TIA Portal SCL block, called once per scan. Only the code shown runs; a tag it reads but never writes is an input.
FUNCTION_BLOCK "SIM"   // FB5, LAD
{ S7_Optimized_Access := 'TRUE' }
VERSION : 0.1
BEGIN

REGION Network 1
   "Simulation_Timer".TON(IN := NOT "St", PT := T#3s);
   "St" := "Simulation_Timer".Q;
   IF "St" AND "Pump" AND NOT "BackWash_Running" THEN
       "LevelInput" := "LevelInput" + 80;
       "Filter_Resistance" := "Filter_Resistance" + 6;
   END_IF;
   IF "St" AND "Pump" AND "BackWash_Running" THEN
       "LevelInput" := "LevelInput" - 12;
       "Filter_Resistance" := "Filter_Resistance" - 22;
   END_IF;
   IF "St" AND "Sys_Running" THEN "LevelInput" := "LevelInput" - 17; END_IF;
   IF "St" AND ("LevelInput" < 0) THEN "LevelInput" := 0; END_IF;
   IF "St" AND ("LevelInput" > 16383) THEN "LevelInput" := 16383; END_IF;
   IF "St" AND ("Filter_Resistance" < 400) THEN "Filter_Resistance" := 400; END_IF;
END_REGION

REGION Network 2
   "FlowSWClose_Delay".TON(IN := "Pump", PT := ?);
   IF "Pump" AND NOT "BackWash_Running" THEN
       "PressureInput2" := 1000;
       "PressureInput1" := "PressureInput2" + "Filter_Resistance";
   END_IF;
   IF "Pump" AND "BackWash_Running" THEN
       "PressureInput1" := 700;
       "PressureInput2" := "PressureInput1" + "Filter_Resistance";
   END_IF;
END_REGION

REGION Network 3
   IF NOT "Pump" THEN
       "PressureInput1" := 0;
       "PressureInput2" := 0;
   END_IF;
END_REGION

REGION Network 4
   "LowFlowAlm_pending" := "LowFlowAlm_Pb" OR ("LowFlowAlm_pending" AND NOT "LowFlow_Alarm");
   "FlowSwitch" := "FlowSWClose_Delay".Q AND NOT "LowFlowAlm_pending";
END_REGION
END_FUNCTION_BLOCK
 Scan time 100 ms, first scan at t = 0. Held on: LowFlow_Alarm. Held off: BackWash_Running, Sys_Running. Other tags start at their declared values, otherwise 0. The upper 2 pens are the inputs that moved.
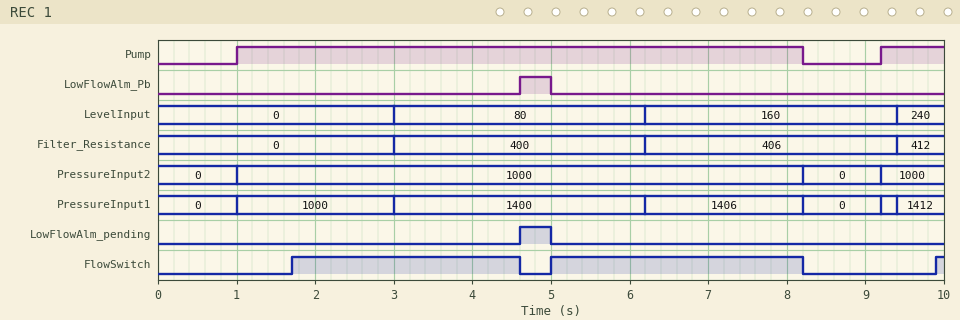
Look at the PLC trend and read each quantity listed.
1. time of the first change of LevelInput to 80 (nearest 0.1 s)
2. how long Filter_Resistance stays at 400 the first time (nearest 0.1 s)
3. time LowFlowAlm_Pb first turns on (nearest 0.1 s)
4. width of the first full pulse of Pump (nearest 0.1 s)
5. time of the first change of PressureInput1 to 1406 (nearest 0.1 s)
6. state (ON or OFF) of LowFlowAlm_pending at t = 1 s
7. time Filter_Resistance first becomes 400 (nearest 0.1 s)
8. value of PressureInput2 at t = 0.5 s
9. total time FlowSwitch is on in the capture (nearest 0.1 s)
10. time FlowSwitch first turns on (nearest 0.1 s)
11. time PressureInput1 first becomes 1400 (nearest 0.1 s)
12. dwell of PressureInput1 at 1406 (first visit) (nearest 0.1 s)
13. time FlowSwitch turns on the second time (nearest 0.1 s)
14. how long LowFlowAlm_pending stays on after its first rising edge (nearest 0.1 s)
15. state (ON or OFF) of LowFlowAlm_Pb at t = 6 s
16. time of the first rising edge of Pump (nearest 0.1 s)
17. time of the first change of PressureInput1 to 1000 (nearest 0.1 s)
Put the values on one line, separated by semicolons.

3.0 s; 3.2 s; 4.6 s; 7.2 s; 6.2 s; OFF; 3.0 s; 0; 6.2 s; 1.7 s; 3.0 s; 2.0 s; 5.0 s; 0.4 s; OFF; 1.0 s; 1.0 s
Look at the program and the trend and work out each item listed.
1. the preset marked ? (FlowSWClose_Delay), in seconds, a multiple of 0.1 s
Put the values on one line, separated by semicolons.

0.7 s
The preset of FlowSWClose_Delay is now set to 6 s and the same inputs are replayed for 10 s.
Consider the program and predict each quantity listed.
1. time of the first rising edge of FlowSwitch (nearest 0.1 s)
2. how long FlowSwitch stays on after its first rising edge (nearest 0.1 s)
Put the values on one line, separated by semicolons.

7.0 s; 1.2 s
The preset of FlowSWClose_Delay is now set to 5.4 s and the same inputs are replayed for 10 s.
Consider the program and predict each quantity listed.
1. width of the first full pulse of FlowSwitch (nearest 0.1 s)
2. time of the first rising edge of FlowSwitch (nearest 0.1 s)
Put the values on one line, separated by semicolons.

1.8 s; 6.4 s
